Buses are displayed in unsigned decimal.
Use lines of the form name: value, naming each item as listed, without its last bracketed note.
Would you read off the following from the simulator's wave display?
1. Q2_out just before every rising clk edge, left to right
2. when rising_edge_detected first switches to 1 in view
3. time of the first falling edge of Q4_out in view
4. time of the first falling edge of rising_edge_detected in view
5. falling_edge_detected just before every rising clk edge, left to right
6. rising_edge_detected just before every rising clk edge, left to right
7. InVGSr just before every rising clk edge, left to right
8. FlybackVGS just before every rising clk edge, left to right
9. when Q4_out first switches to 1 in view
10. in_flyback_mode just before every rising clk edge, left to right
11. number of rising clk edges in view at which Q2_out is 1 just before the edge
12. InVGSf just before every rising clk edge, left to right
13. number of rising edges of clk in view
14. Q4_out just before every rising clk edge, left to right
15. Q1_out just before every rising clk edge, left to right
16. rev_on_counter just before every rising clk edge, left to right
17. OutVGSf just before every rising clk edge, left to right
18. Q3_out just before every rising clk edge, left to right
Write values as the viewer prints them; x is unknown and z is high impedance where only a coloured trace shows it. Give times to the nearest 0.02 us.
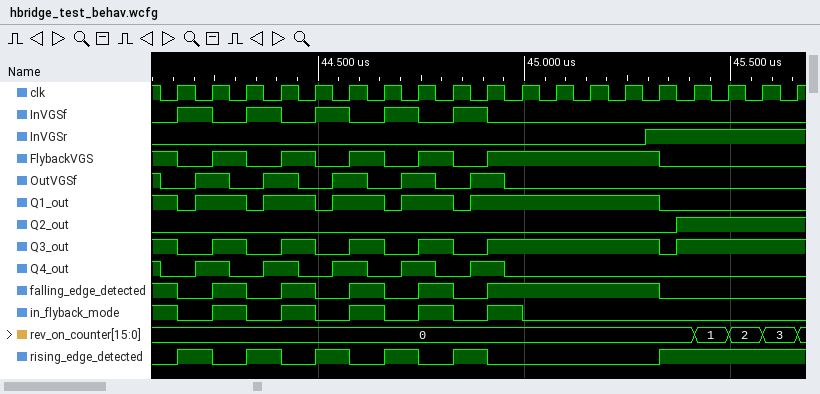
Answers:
Q2_out just before every rising clk edge, left to right: 0 0 0 0 0 0 0 0 0 0 0 0 0 0 0 1 1 1 1
when rising_edge_detected first switches to 1 in view: 44.16 us
time of the first falling edge of Q4_out in view: 44.12 us
time of the first falling edge of rising_edge_detected in view: 44.24 us
falling_edge_detected just before every rising clk edge, left to right: 1 0 1 0 1 0 1 0 1 0 1 1 1 1 1 0 0 0 0
rising_edge_detected just before every rising clk edge, left to right: 0 1 0 1 0 1 0 1 0 1 0 0 0 0 0 1 1 1 1
InVGSr just before every rising clk edge, left to right: 0 0 0 0 0 0 0 0 0 0 0 0 0 0 1 1 1 1 1
FlybackVGS just before every rising clk edge, left to right: 1 0 1 0 1 0 1 0 1 0 1 1 1 1 1 0 0 0 0
when Q4_out first switches to 1 in view: 44.2 us
in_flyback_mode just before every rising clk edge, left to right: 1 0 1 0 1 0 1 0 1 0 1 0 0 0 0 0 0 0 0
number of rising clk edges in view at which Q2_out is 1 just before the edge: 4
InVGSf just before every rising clk edge, left to right: 0 1 0 1 0 1 0 1 0 1 0 0 0 0 0 0 0 0 0
number of rising edges of clk in view: 19
Q4_out just before every rising clk edge, left to right: 0 1 0 1 0 1 0 1 0 1 0 0 0 0 0 0 0 0 0
Q1_out just before every rising clk edge, left to right: 1 1 1 1 1 1 1 1 1 1 1 1 1 1 1 0 0 0 0
rev_on_counter just before every rising clk edge, left to right: 0, 0, 0, 0, 0, 0, 0, 0, 0, 0, 0, 0, 0, 0, 0, 0, 1, 2, 3
OutVGSf just before every rising clk edge, left to right: 0 1 0 1 0 1 0 1 0 1 0 0 0 0 0 0 0 0 0
Q3_out just before every rising clk edge, left to right: 1 0 1 0 1 0 1 0 1 0 1 1 1 1 1 1 1 1 1
